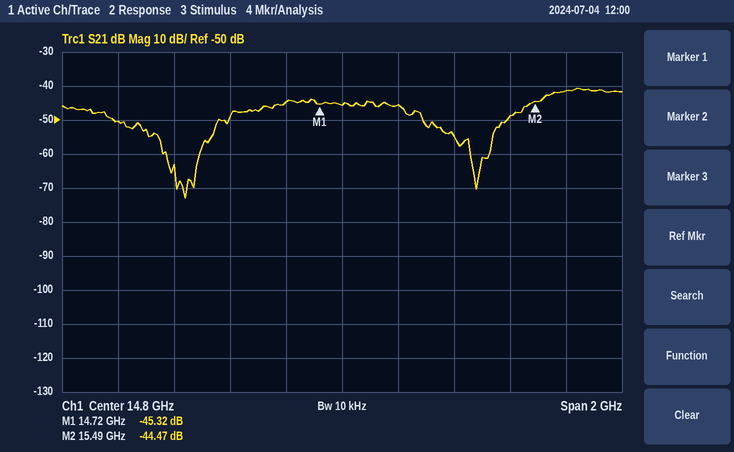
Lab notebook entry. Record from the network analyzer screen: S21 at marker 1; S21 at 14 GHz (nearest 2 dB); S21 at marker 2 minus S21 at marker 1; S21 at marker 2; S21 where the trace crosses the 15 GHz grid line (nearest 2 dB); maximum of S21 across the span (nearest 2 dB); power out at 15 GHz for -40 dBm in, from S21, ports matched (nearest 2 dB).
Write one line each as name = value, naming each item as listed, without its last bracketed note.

S21 at marker 1 = -45.32 dB
S21 at 14 GHz = -50 dB
S21 at marker 2 minus S21 at marker 1 = 0.85 dB
S21 at marker 2 = -44.47 dB
S21 where the trace crosses the 15 GHz grid line = -46 dB
maximum of S21 across the span = -40 dB
power out at 15 GHz for -40 dBm in, from S21, ports matched = -86 dBm
